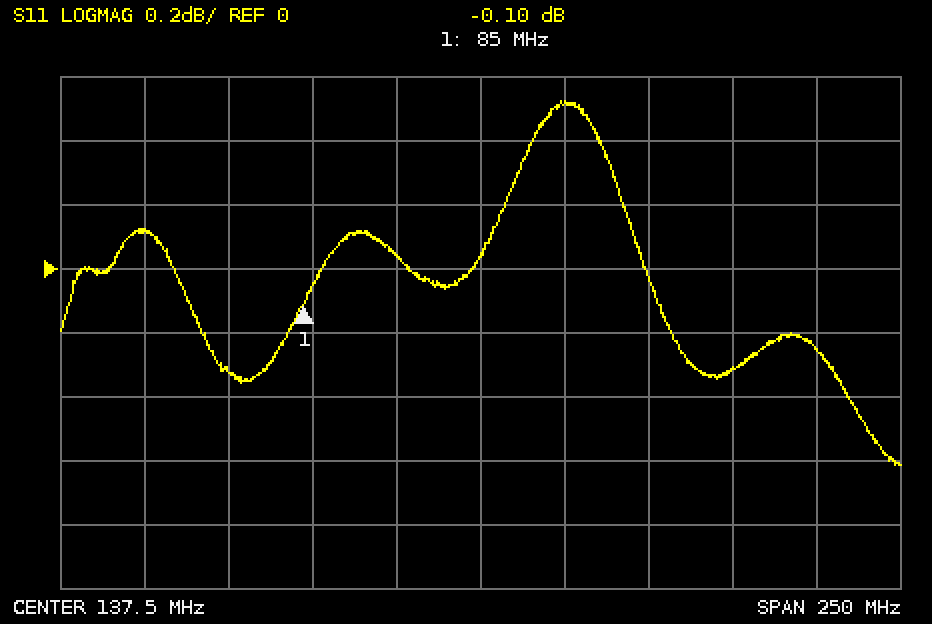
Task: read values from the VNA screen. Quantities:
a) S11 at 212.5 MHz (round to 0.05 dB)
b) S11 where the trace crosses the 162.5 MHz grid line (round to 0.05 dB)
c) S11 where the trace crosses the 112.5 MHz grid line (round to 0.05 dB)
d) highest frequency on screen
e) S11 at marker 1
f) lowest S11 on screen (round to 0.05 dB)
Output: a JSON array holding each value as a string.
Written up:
["-0.30 dB", "0.50 dB", "0.05 dB", "262.5 MHz", "-0.10 dB", "-0.60 dB"]
